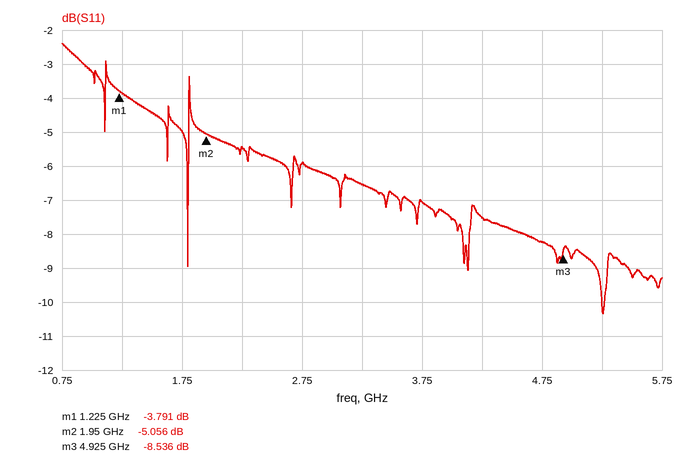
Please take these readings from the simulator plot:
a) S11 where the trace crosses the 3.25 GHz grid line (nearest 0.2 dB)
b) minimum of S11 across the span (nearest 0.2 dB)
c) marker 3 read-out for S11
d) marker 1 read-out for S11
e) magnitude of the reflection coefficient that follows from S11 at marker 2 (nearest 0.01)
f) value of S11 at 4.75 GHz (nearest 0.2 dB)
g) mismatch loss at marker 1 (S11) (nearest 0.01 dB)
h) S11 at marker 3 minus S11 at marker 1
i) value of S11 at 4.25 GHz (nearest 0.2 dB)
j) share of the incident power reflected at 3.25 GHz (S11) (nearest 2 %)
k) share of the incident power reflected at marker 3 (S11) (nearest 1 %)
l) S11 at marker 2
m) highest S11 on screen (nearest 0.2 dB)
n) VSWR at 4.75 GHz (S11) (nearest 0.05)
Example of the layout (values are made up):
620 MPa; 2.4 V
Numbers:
-6.6 dB; -10.4 dB; -8.536 dB; -3.791 dB; 0.56; -8.2 dB; 2.35 dB; -4.745 dB; -7.6 dB; 22 %; 14 %; -5.056 dB; -2.4 dB; 2.25
